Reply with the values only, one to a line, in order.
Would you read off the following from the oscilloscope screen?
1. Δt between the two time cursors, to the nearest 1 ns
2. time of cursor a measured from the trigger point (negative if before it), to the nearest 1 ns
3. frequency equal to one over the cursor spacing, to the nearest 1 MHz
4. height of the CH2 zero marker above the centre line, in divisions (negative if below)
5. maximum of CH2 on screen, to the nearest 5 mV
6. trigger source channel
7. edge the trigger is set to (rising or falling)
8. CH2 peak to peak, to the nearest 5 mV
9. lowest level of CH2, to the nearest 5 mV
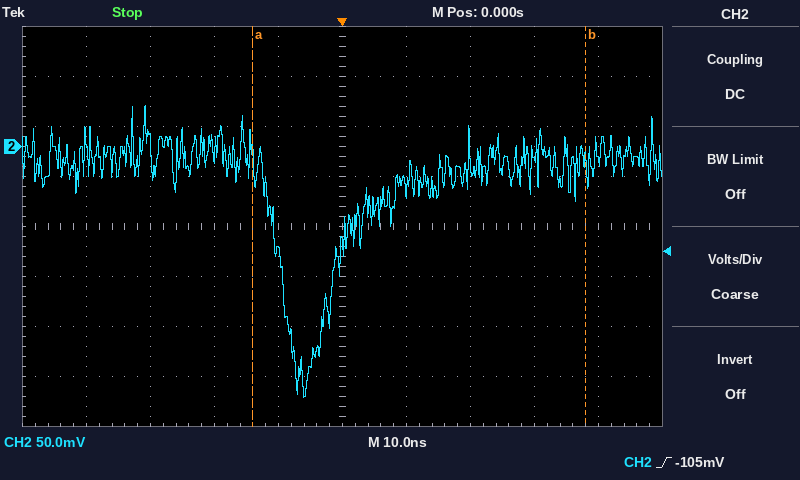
52 ns
-14 ns
19 MHz
+1.6 div
40 mV
CH2
rising
290 mV
-250 mV
